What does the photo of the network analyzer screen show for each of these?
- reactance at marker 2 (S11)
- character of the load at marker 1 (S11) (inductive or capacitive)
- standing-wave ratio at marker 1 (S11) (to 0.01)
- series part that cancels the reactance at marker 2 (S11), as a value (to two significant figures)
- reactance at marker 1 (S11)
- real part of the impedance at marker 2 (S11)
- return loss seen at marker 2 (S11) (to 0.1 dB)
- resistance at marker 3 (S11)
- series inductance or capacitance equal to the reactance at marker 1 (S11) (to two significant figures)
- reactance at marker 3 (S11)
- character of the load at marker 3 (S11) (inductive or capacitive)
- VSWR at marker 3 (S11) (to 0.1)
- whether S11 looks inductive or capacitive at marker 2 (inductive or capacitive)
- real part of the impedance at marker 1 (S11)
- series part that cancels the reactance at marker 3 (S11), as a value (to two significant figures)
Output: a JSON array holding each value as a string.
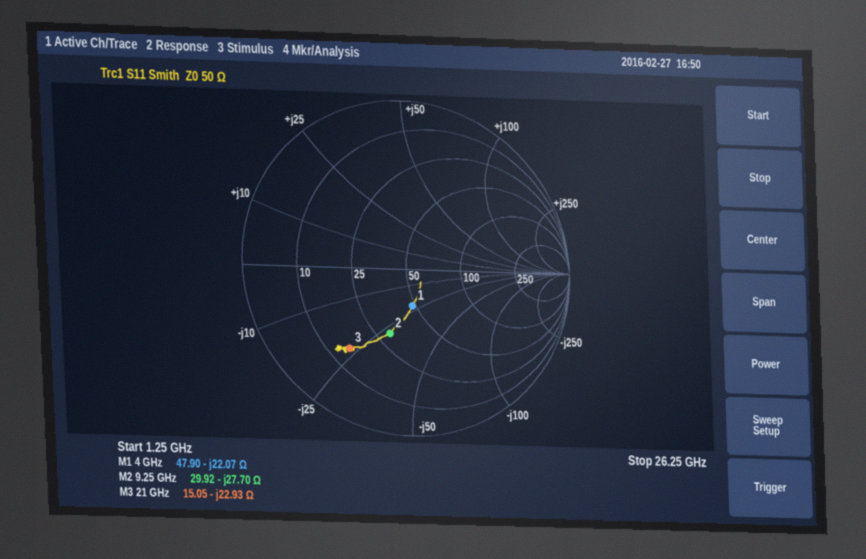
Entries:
["-27.70 Ω", "capacitive", "1.57", "480 pH", "-22.07 Ω", "29.92 Ω", "7.9 dB", "15.05 Ω", "1.8 pF", "-22.93 Ω", "capacitive", "4.1", "capacitive", "47.90 Ω", "170 pH"]
